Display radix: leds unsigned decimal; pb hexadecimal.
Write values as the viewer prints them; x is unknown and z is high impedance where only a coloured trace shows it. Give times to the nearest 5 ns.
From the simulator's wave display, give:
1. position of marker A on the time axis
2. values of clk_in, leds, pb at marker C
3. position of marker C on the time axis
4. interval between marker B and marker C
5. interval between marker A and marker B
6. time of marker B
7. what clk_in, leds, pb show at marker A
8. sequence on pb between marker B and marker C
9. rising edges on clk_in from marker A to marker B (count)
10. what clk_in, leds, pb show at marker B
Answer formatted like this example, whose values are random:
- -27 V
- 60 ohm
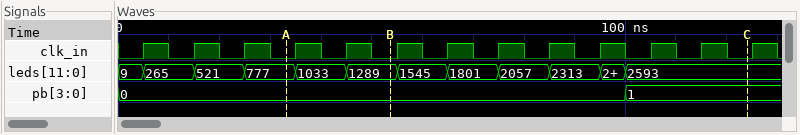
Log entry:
- 35 ns
- clk_in=0, leds=2593, pb=1
- 125 ns
- 70 ns
- 20 ns
- 55 ns
- clk_in=0, leds=777, pb=0
- 0, 1
- 2
- clk_in=0, leds=1289, pb=0
